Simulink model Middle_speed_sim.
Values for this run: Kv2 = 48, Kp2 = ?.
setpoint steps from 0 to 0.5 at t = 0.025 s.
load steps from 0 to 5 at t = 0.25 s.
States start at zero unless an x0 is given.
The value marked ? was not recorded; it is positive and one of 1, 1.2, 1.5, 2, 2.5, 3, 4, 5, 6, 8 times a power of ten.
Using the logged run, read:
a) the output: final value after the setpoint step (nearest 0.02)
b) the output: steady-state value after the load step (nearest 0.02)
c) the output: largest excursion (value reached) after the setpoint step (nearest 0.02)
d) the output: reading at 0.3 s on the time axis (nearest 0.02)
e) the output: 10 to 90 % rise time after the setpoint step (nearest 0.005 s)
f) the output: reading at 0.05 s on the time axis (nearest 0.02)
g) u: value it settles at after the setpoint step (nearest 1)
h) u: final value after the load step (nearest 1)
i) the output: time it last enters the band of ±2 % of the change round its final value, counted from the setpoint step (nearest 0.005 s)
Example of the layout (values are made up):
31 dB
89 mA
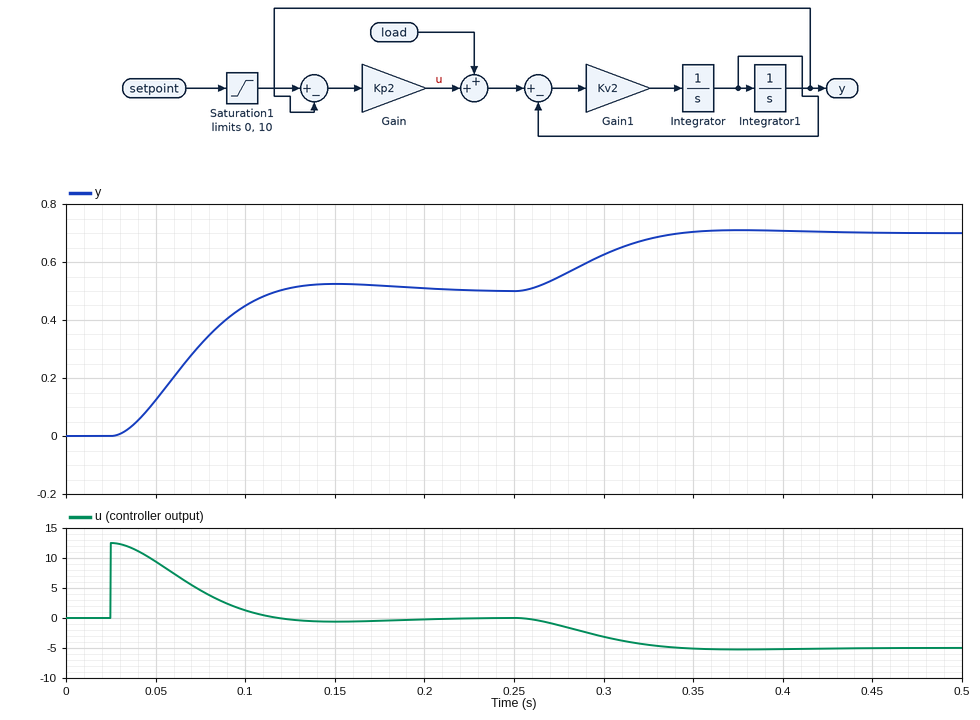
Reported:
0.50
0.70
0.52
0.62
0.060 s
0.12
0
-5
0.175 s
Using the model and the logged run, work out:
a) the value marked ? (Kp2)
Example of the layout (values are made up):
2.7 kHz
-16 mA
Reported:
25
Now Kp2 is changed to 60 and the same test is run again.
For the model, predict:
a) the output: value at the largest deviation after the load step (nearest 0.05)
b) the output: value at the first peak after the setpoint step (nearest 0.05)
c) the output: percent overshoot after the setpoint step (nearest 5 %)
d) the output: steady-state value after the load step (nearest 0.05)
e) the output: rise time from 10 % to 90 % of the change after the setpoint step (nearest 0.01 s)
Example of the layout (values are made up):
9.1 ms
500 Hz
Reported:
0.60
0.60
20 %
0.60
0.03 s
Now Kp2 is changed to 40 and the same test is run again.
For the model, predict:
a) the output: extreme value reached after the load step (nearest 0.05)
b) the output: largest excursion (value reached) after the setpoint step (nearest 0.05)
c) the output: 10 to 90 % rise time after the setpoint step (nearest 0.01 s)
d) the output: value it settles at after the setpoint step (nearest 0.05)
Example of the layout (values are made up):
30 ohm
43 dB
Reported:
0.65
0.55
0.04 s
0.50
